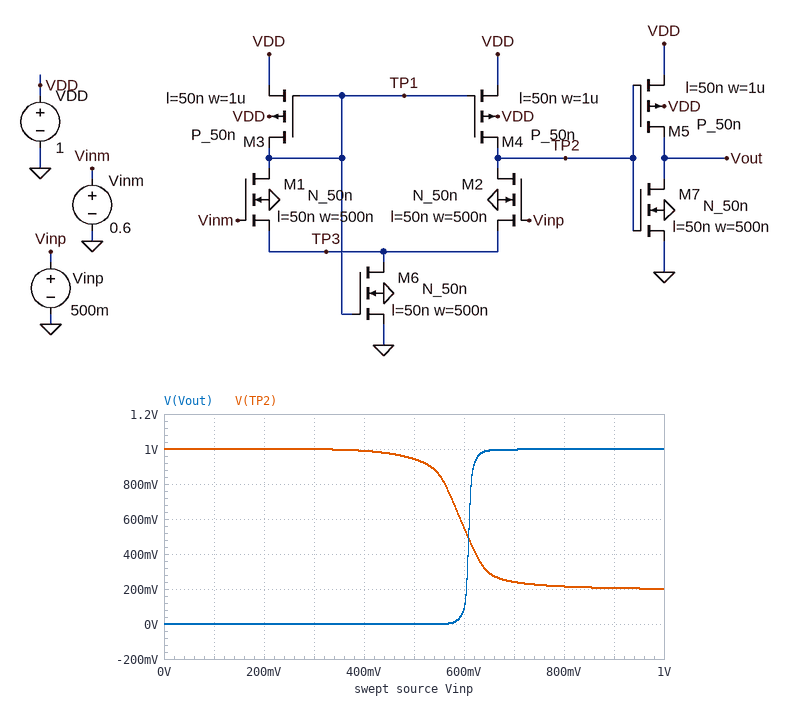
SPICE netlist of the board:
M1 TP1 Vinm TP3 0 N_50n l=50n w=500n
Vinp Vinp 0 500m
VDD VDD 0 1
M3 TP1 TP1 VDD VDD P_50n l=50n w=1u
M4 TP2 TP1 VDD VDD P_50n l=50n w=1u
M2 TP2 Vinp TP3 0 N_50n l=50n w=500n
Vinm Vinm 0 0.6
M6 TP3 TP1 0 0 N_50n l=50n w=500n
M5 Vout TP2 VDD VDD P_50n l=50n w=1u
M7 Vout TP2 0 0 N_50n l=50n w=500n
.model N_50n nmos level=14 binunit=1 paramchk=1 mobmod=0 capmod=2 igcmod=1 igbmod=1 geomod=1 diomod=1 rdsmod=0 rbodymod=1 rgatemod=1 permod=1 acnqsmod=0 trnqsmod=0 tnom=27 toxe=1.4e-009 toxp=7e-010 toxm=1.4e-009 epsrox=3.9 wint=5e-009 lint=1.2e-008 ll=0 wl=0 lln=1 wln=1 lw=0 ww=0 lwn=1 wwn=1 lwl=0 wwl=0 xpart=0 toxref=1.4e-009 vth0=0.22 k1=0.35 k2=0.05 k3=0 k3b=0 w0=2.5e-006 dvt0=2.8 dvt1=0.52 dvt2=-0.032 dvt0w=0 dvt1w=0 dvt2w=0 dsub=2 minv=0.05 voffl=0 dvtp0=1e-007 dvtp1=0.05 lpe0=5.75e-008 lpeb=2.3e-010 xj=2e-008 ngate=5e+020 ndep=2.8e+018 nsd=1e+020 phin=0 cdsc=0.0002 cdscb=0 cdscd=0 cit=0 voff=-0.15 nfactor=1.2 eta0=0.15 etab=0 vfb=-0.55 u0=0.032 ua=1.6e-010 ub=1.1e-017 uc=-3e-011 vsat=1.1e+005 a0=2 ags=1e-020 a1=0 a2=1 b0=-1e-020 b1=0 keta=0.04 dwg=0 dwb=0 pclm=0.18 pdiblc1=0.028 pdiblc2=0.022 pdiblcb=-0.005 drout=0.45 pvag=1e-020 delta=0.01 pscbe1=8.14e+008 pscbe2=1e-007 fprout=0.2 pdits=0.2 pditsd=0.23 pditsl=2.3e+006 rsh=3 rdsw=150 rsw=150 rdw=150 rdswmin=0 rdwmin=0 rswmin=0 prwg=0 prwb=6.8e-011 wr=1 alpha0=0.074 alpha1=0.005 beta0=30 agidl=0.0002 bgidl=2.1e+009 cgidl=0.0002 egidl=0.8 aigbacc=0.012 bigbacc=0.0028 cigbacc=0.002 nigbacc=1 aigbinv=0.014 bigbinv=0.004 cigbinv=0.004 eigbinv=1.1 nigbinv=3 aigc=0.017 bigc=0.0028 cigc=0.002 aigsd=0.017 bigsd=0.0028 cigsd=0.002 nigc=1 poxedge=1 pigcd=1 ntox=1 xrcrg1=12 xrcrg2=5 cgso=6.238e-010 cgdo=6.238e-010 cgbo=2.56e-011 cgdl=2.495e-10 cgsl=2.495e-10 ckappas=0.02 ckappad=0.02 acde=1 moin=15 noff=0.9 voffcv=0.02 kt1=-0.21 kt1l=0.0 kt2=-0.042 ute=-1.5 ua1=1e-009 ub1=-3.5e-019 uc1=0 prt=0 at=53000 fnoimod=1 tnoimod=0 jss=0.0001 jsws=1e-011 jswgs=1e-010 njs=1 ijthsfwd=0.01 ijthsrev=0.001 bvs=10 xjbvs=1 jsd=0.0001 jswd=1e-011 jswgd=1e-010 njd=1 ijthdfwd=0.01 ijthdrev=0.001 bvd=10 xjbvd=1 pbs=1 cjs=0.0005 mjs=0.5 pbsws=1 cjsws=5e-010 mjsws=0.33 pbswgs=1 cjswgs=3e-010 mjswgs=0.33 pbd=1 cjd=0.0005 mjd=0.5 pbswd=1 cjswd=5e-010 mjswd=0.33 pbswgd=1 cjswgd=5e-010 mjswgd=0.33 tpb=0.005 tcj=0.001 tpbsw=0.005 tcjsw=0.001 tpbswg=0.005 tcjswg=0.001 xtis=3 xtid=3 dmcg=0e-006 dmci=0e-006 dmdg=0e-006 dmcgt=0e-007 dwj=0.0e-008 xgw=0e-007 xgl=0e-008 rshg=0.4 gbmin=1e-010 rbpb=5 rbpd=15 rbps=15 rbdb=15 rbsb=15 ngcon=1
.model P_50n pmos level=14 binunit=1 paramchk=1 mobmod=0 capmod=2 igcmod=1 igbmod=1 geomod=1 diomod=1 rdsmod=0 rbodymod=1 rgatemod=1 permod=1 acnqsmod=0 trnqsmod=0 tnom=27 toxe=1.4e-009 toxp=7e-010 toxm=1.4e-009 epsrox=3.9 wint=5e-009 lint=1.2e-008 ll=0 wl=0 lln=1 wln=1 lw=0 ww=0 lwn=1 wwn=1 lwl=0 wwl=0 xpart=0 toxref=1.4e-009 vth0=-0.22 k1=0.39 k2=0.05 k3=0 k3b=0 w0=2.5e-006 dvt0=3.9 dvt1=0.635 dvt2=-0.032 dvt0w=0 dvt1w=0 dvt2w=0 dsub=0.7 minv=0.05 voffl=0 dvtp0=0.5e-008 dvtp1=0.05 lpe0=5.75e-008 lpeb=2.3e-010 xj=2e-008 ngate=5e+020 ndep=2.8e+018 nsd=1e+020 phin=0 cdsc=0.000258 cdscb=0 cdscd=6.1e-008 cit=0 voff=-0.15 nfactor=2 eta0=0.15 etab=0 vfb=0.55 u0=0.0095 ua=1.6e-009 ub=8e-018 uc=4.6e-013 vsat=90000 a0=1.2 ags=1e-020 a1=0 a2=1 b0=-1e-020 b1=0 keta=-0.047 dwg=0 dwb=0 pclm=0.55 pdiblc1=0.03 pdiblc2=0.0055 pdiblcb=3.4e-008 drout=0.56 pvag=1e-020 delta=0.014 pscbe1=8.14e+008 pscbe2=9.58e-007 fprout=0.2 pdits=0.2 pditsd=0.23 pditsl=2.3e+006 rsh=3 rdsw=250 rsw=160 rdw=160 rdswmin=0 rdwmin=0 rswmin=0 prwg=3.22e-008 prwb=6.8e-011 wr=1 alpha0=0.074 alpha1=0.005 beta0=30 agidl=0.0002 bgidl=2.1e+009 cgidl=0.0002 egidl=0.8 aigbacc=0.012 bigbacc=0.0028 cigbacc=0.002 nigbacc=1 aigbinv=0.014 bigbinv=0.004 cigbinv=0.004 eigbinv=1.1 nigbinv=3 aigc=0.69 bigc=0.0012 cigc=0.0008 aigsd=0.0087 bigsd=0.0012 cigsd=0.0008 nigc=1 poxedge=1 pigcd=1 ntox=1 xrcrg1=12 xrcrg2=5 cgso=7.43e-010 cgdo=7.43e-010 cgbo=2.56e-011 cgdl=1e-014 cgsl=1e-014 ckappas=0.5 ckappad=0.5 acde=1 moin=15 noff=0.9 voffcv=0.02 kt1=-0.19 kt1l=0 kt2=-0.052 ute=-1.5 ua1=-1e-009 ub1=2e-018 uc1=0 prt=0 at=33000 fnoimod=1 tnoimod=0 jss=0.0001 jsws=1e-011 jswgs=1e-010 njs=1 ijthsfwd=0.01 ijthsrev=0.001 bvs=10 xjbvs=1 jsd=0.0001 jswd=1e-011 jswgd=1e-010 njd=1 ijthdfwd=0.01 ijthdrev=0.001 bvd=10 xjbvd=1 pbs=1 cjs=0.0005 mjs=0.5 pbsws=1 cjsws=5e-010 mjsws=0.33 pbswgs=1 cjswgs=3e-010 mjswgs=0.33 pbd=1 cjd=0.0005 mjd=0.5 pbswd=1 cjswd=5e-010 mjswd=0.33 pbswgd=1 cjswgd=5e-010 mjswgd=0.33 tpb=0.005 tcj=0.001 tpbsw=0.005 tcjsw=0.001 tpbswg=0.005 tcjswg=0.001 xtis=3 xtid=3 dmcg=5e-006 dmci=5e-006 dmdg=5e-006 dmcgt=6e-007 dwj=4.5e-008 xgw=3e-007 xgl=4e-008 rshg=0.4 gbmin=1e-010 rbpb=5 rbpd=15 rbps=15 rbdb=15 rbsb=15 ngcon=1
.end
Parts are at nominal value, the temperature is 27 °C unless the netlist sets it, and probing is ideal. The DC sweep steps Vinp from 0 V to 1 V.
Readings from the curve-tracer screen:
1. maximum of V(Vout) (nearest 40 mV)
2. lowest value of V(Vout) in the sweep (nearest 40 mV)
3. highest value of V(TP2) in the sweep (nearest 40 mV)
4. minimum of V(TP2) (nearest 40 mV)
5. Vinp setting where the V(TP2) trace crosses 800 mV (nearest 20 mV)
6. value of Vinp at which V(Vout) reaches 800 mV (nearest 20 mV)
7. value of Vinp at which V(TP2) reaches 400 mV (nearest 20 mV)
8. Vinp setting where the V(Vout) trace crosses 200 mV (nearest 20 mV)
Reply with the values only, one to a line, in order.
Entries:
1.00 V
0 V
1.00 V
200 mV
560 mV
620 mV
620 mV
600 mV
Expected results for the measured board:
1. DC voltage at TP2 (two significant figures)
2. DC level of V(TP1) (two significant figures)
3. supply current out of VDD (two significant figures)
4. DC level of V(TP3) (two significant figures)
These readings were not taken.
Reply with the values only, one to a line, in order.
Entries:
940 mV
530 mV
47 µA
130 mV
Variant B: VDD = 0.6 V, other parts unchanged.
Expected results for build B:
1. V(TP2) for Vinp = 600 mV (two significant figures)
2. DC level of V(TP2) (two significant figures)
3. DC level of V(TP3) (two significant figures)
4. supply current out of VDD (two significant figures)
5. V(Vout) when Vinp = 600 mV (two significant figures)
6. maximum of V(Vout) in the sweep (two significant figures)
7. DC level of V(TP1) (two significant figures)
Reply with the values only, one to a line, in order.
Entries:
310 mV
580 mV
260 mV
3.2 µA
68 mV
530 mV
300 mV
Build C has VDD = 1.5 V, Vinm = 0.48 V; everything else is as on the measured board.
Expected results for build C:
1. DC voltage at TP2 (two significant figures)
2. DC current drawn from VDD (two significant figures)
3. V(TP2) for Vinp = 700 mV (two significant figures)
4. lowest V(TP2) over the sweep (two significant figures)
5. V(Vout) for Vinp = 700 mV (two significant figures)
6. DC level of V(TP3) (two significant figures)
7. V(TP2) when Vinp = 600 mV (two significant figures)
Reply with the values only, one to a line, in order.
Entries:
890 mV
200 µA
170 mV
140 mV
1.5 V
67 mV
260 mV
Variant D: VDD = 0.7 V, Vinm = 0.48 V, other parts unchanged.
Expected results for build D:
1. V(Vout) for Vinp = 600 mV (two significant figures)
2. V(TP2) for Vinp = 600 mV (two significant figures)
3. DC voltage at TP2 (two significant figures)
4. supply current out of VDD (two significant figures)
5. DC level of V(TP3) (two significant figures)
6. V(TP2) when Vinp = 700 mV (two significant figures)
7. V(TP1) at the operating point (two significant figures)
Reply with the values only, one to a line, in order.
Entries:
700 mV
170 mV
250 mV
11 µA
150 mV
160 mV
370 mV
